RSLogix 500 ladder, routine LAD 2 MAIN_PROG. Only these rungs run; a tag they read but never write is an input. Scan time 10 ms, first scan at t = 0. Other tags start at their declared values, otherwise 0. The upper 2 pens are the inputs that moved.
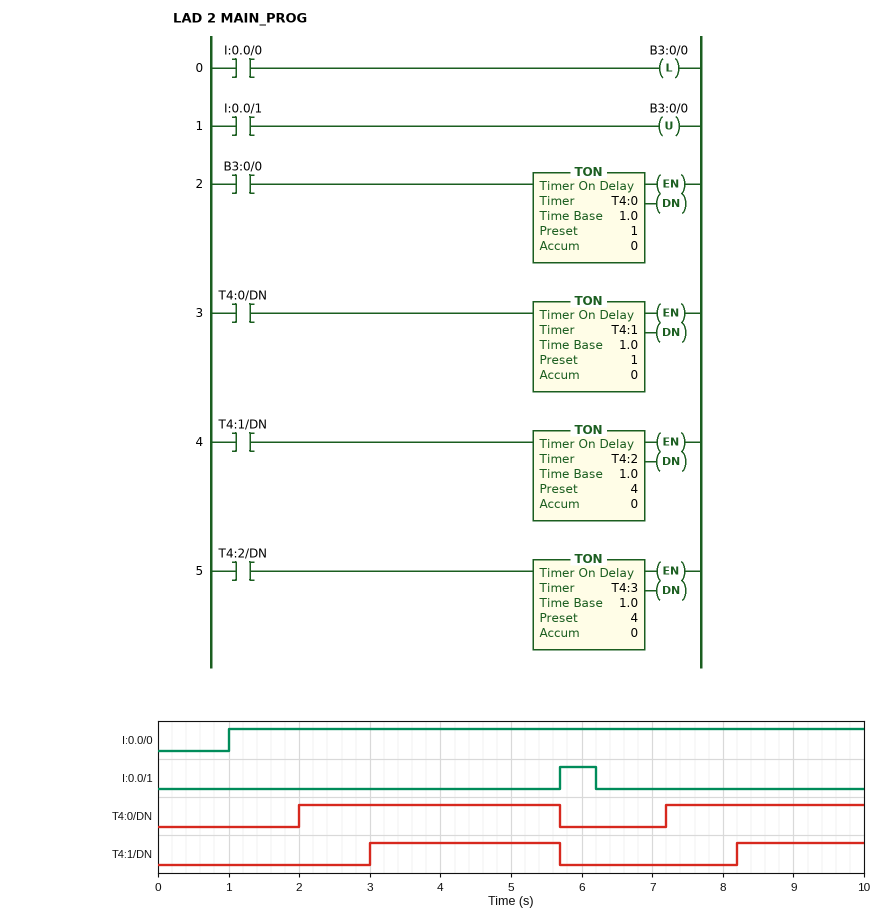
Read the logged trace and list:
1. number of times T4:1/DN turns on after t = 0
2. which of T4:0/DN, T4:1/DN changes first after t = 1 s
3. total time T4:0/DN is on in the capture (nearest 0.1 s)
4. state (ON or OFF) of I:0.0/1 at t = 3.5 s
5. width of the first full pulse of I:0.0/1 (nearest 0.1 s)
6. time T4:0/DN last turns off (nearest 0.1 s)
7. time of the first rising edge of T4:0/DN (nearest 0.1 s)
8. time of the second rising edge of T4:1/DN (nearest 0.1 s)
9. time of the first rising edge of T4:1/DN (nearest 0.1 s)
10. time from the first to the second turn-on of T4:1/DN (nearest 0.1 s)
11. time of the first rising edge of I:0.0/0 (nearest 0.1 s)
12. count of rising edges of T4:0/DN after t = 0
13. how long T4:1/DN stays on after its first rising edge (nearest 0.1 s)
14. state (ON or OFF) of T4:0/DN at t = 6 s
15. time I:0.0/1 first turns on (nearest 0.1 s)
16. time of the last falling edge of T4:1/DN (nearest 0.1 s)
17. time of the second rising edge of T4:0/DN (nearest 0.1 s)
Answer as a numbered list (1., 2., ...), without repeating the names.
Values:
1. 2
2. T4:0/DN
3. 6.5 s
4. OFF
5. 0.5 s
6. 5.7 s
7. 2.0 s
8. 8.2 s
9. 3.0 s
10. 5.2 s
11. 1.0 s
12. 2
13. 2.7 s
14. OFF
15. 5.7 s
16. 5.7 s
17. 7.2 s
